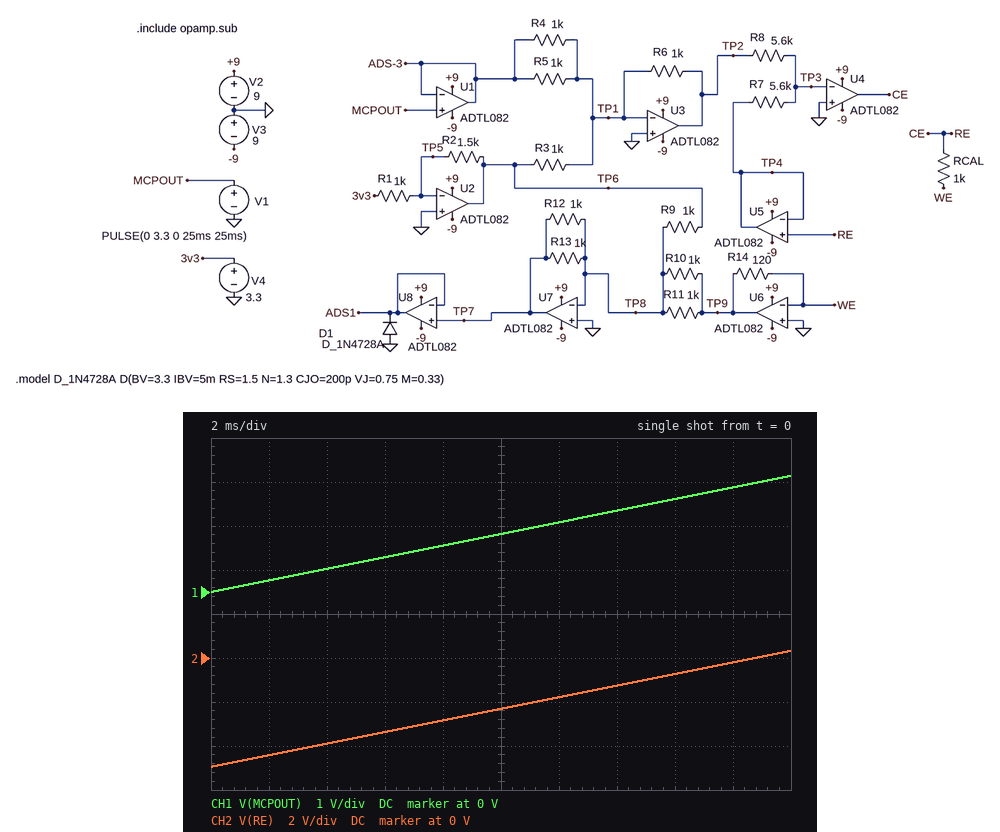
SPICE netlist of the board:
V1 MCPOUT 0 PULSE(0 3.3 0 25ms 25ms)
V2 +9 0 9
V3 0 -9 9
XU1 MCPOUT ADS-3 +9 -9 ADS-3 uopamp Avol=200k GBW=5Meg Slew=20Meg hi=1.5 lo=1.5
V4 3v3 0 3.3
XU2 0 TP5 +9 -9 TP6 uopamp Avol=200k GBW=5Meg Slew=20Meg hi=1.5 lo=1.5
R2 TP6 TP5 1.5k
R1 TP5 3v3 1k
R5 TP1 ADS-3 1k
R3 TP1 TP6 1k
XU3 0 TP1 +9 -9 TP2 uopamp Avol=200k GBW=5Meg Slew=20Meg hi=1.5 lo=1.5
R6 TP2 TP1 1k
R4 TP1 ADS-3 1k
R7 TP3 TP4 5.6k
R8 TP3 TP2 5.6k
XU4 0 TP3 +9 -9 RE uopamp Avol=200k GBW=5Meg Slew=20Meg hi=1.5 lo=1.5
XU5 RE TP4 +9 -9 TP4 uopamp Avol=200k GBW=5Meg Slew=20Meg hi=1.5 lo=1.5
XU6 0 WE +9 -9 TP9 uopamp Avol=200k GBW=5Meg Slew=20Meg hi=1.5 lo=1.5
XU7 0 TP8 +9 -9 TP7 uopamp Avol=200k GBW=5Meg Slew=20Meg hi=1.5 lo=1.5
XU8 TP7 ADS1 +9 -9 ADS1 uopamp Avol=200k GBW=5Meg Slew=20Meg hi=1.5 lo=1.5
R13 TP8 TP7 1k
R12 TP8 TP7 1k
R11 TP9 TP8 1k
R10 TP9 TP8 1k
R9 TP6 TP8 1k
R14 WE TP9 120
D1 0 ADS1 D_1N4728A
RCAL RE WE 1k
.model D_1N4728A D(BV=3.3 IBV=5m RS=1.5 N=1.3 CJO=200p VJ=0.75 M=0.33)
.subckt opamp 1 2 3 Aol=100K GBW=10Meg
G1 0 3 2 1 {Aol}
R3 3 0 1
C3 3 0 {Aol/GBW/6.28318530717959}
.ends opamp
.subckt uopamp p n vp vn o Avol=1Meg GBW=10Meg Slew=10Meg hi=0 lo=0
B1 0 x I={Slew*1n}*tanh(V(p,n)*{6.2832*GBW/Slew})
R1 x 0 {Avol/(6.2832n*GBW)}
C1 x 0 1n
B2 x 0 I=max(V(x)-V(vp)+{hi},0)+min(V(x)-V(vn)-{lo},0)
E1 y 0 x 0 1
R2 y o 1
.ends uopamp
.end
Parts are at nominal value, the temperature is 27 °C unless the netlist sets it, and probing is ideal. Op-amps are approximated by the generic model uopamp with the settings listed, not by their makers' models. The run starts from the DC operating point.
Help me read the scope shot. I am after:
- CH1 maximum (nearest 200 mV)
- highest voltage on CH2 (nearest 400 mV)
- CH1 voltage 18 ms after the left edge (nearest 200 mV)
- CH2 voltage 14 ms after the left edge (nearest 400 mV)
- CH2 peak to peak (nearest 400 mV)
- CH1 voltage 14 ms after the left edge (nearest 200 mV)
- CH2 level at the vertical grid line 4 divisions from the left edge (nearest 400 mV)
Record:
2.6 V
400 mV
2.4 V
-1.2 V
5.2 V
1.8 V
-2.8 V
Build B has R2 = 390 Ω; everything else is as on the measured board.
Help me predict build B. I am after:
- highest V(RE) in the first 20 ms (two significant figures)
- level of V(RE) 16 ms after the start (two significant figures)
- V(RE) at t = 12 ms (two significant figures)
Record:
4.0 V
2.9 V
1.9 V
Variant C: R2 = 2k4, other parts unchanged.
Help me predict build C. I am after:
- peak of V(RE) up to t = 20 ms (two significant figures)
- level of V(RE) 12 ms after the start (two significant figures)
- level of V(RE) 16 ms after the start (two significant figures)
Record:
-2.2 V
-4.3 V
-3.3 V
